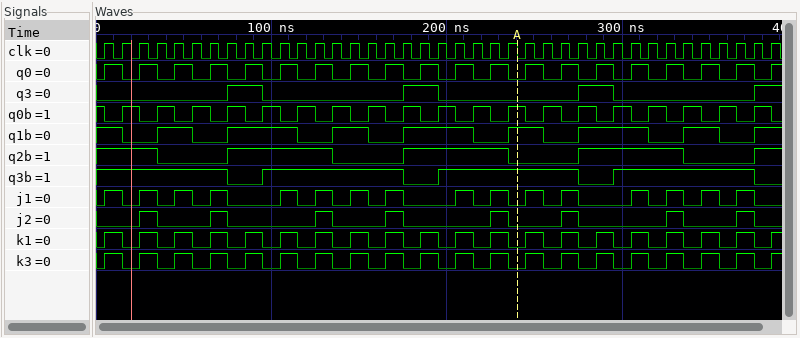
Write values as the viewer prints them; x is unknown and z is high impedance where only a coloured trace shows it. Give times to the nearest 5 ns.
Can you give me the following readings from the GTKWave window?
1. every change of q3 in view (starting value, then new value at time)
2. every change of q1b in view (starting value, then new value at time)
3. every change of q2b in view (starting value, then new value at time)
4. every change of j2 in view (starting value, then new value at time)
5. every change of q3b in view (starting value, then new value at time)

0, 1 at 75 ns, 0 at 95 ns, 1 at 175 ns, 0 at 195 ns, 1 at 275 ns, 0 at 295 ns, 1 at 375 ns
1, 0 at 15 ns, 1 at 35 ns, 0 at 55 ns, 1 at 75 ns, 0 at 115 ns, 1 at 135 ns, 0 at 155 ns, 1 at 175 ns, 0 at 215 ns, 1 at 235 ns, 0 at 255 ns, 1 at 275 ns, 0 at 315 ns, 1 at 335 ns, 0 at 355 ns, 1 at 375 ns
1, 0 at 35 ns, 1 at 75 ns, 0 at 135 ns, 1 at 175 ns, 0 at 235 ns, 1 at 275 ns, 0 at 335 ns, 1 at 375 ns
0, 1 at 25 ns, 0 at 35 ns, 1 at 65 ns, 0 at 75 ns, 1 at 125 ns, 0 at 135 ns, 1 at 165 ns, 0 at 175 ns, 1 at 225 ns, 0 at 235 ns, 1 at 265 ns, 0 at 275 ns, 1 at 325 ns, 0 at 335 ns, 1 at 365 ns, 0 at 375 ns
1, 0 at 75 ns, 1 at 95 ns, 0 at 175 ns, 1 at 195 ns, 0 at 275 ns, 1 at 295 ns, 0 at 375 ns
